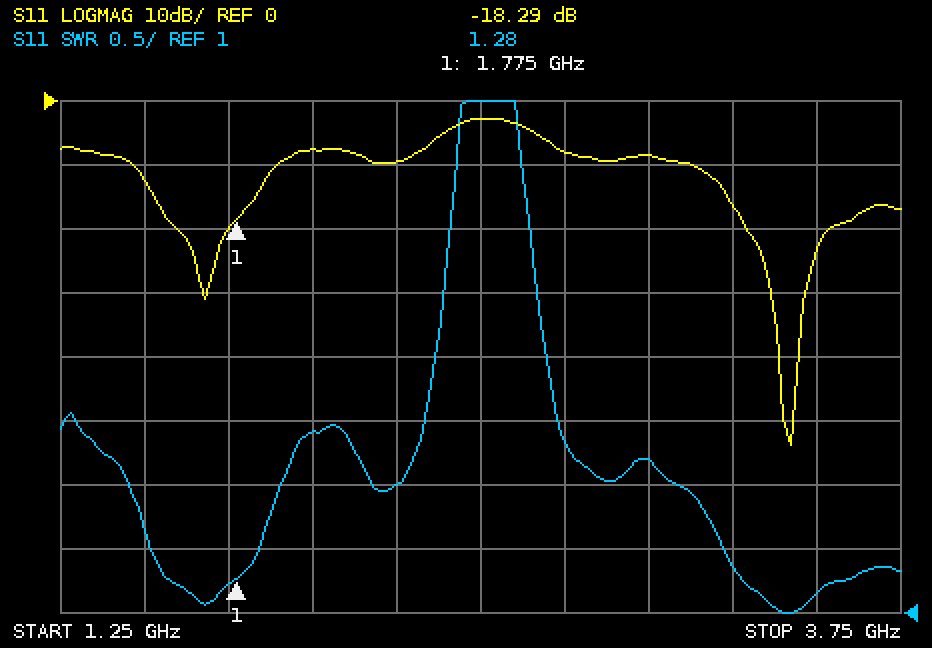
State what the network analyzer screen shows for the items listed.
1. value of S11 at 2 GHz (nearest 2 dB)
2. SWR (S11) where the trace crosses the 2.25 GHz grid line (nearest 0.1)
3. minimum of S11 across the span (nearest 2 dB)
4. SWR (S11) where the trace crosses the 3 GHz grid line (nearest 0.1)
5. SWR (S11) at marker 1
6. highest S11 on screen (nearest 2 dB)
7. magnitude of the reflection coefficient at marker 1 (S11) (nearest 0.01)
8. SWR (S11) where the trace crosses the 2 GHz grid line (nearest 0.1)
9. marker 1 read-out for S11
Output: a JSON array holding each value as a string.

["-8 dB", "2.0", "-54 dB", "2.2", "1.28", "-2 dB", "0.12", "2.4", "-18.29 dB"]
